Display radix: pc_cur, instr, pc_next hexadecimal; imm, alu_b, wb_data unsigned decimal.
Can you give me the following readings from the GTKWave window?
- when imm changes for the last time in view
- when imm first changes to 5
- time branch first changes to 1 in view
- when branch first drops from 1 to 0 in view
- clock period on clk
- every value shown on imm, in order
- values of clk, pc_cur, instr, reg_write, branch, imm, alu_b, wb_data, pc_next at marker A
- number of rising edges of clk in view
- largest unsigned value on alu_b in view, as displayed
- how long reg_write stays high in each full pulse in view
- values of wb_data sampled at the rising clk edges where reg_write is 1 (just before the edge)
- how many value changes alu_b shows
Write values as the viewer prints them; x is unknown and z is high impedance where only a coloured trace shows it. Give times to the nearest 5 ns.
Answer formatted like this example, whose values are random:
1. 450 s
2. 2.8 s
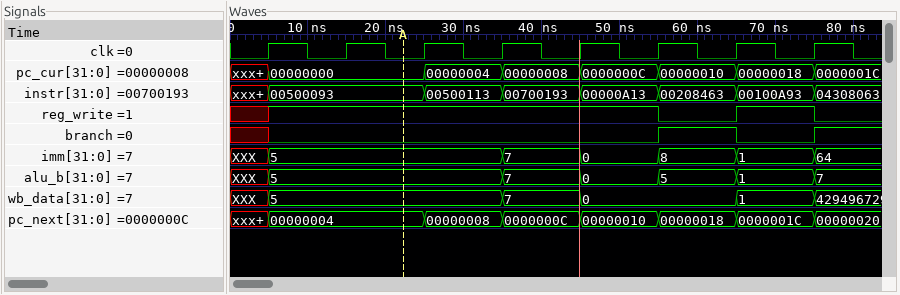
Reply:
1. 75 ns
2. 5 ns
3. 55 ns
4. 65 ns
5. 10 ns
6. XXX, 5, 7, 0, 8, 1, 64
7. clk=0, pc_cur=00000000, instr=00500093, reg_write=1, branch=0, imm=5, alu_b=5, wb_data=5, pc_next=00000004
8. 8
9. 7
10. 10 ns
11. 5, 5, 5, 7, 0, 1
12. 6
